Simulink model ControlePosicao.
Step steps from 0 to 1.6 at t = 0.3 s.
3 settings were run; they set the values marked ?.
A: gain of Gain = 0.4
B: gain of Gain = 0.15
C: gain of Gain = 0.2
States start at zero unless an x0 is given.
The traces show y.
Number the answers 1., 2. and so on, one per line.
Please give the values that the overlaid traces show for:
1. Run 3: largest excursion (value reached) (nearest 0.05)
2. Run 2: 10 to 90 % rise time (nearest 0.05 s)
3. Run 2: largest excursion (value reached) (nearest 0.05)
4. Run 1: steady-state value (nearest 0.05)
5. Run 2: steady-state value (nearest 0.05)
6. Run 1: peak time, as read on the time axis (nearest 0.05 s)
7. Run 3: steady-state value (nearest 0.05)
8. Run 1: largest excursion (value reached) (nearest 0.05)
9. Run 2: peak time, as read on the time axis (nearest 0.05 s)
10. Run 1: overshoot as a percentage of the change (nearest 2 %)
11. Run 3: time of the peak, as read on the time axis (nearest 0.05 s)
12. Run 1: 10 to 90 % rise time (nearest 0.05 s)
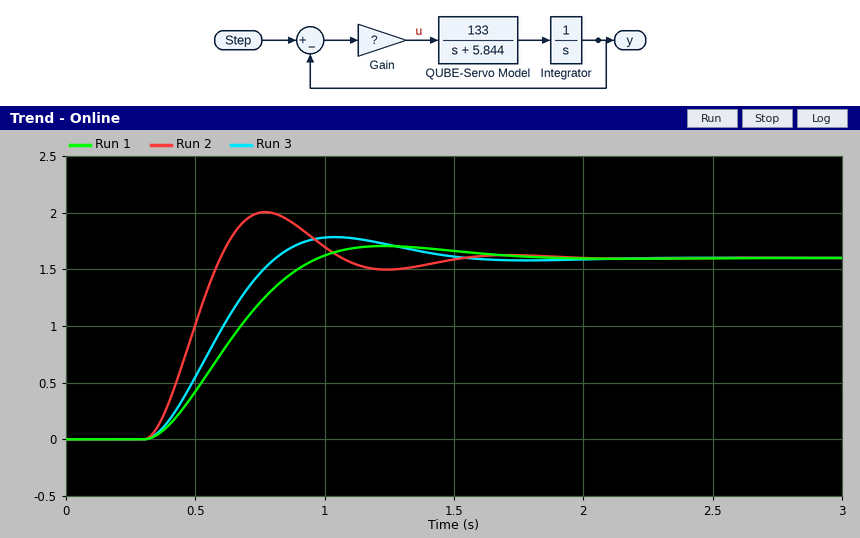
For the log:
1. 1.80
2. 0.20 s
3. 2.00
4. 1.60
5. 1.60
6. 1.25 s
7. 1.60
8. 1.70
9. 0.75 s
10. 6 %
11. 1.05 s
12. 0.45 s
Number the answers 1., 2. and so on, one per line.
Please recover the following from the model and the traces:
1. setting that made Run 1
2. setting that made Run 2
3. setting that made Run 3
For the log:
1. B
2. A
3. C
